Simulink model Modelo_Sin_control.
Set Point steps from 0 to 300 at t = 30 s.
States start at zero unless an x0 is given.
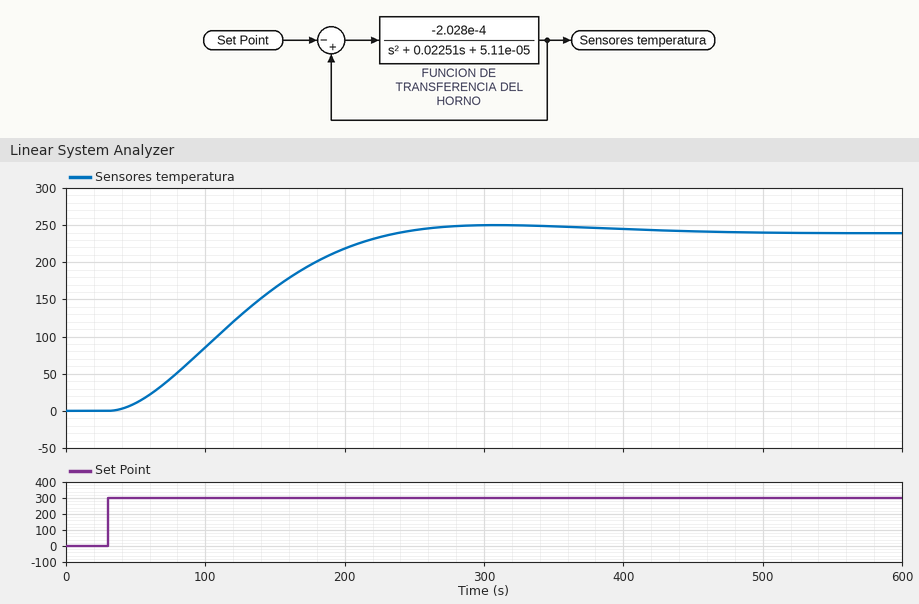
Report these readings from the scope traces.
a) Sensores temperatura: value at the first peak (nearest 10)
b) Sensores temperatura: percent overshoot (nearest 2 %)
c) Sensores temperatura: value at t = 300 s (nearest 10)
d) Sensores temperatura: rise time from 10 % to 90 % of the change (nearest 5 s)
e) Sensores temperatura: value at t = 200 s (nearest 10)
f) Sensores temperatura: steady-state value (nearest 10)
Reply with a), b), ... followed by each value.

a) 250
b) 4 %
c) 250
d) 135 s
e) 220
f) 240
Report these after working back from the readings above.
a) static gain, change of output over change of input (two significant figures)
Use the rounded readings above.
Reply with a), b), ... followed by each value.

a) 0.80
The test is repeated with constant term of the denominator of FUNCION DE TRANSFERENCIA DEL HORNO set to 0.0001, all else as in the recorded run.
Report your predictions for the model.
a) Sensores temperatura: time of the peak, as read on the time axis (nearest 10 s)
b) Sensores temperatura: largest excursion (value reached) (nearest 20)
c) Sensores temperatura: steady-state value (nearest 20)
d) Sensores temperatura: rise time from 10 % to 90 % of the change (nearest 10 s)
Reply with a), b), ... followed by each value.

a) 270 s
b) 220
c) 200
d) 110 s
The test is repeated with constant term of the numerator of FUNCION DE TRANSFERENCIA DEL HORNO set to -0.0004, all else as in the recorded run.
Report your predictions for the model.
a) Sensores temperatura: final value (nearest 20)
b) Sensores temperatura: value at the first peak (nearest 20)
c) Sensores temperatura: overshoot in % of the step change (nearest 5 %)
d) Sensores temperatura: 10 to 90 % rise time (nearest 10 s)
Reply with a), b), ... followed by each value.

a) 260
b) 300
c) 15 %
d) 80 s
